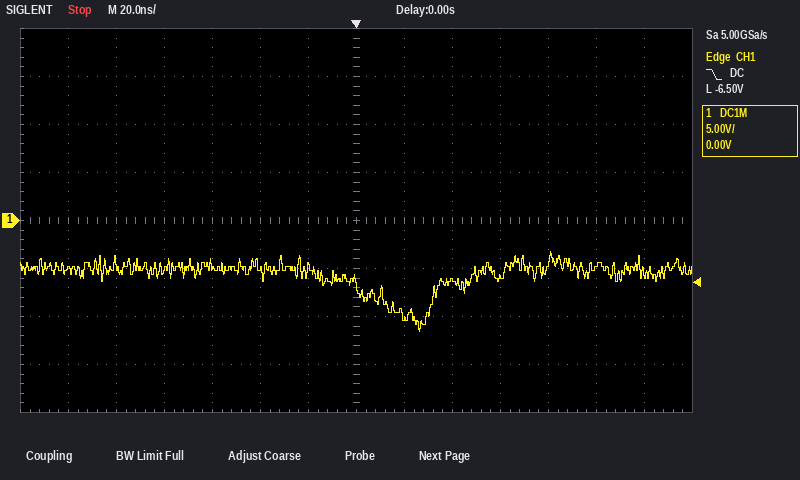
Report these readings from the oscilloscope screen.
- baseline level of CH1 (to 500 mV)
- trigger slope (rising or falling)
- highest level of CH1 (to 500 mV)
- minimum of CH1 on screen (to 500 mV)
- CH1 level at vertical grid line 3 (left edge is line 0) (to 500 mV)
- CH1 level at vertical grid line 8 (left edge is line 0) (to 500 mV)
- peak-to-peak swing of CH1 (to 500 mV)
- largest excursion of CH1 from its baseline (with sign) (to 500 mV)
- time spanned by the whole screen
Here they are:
-5.0 V
falling
-3.0 V
-11.5 V
-5.0 V
-10.0 V
8.5 V
-6.5 V
280 ns
